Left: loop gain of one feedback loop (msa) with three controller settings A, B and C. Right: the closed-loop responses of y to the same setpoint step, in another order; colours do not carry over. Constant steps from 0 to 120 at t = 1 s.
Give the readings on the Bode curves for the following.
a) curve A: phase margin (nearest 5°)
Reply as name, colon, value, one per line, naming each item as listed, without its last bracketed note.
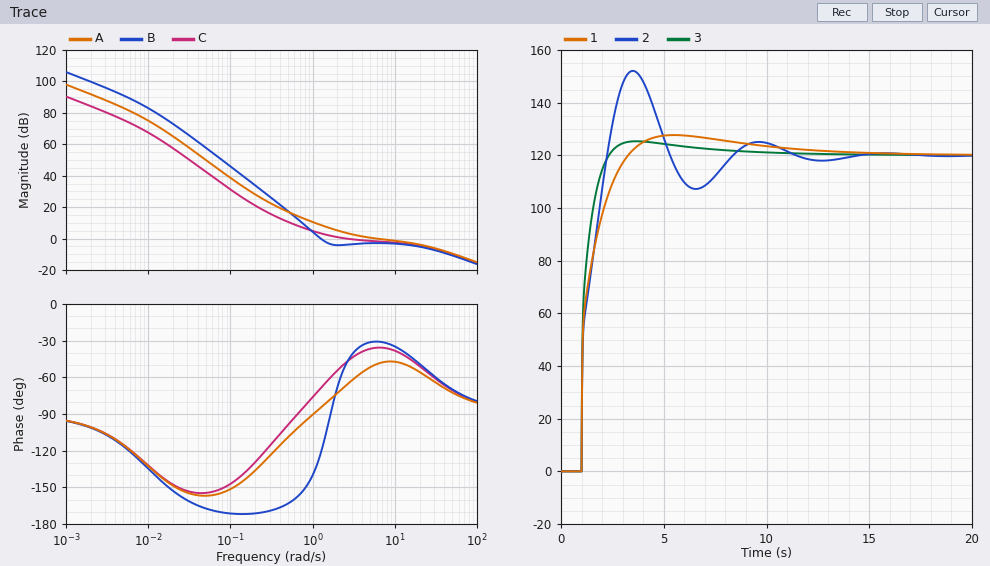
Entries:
curve A: phase margin: 130°
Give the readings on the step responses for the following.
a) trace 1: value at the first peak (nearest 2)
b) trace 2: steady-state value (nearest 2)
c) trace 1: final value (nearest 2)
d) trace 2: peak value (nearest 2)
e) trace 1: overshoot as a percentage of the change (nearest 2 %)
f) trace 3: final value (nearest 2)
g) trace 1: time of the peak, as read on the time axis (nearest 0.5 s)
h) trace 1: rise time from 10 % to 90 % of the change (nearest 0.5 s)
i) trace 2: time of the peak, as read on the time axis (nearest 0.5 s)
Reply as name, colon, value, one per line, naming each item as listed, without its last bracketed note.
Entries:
trace 1: value at the first peak: 128
trace 2: steady-state value: 120
trace 1: final value: 120
trace 2: peak value: 152
trace 1: overshoot as a percentage of the change: 6 %
trace 3: final value: 120
trace 1: time of the peak, as read on the time axis: 5.5 s
trace 1: rise time from 10 % to 90 % of the change: 1.5 s
trace 2: time of the peak, as read on the time axis: 3.5 s
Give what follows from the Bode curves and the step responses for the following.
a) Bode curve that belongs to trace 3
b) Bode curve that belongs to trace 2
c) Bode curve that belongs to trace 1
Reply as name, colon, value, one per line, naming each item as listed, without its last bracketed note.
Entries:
Bode curve that belongs to trace 3: A
Bode curve that belongs to trace 2: B
Bode curve that belongs to trace 1: C
